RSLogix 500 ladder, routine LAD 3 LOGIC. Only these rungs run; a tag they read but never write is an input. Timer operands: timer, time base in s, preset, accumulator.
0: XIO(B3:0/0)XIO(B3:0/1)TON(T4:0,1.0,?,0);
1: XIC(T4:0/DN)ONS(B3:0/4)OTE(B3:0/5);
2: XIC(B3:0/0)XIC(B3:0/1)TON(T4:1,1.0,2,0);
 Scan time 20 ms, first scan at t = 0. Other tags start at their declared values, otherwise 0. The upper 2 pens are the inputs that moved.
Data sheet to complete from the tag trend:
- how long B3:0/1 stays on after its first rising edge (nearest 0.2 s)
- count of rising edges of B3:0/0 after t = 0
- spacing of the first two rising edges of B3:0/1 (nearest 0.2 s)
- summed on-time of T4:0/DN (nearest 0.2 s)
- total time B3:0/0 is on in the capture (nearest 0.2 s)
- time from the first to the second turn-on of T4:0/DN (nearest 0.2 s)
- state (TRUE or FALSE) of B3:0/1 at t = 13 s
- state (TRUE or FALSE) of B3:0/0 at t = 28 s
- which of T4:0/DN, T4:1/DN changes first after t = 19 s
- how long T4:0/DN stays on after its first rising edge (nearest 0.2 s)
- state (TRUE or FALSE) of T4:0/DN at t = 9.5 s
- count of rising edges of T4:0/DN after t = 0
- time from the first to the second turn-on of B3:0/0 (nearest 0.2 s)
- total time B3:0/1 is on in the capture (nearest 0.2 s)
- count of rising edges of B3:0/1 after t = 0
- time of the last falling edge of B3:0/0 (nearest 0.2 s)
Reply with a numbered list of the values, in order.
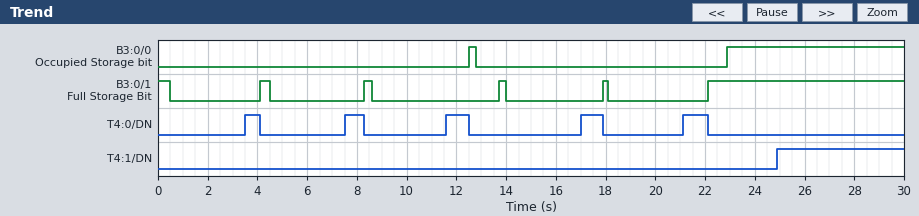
1. 0.4 s
2. 2
3. 4.2 s
4. 4.2 s
5. 7.4 s
6. 4.0 s
7. FALSE
8. TRUE
9. T4:0/DN
10. 0.6 s
11. FALSE
12. 5
13. 10.4 s
14. 9.6 s
15. 5
16. 12.8 s
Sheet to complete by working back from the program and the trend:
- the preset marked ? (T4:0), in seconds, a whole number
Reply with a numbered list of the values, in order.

1. 3 s
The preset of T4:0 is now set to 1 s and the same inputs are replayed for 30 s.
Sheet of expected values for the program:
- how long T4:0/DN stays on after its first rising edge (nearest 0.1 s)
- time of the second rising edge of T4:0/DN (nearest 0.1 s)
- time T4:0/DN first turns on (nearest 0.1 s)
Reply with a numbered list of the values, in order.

1. 2.6 s
2. 5.5 s
3. 1.5 s
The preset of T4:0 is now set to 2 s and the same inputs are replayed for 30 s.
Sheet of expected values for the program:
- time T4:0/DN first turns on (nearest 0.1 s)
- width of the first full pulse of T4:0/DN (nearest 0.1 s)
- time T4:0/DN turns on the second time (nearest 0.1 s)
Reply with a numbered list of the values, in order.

1. 2.5 s
2. 1.6 s
3. 6.5 s
